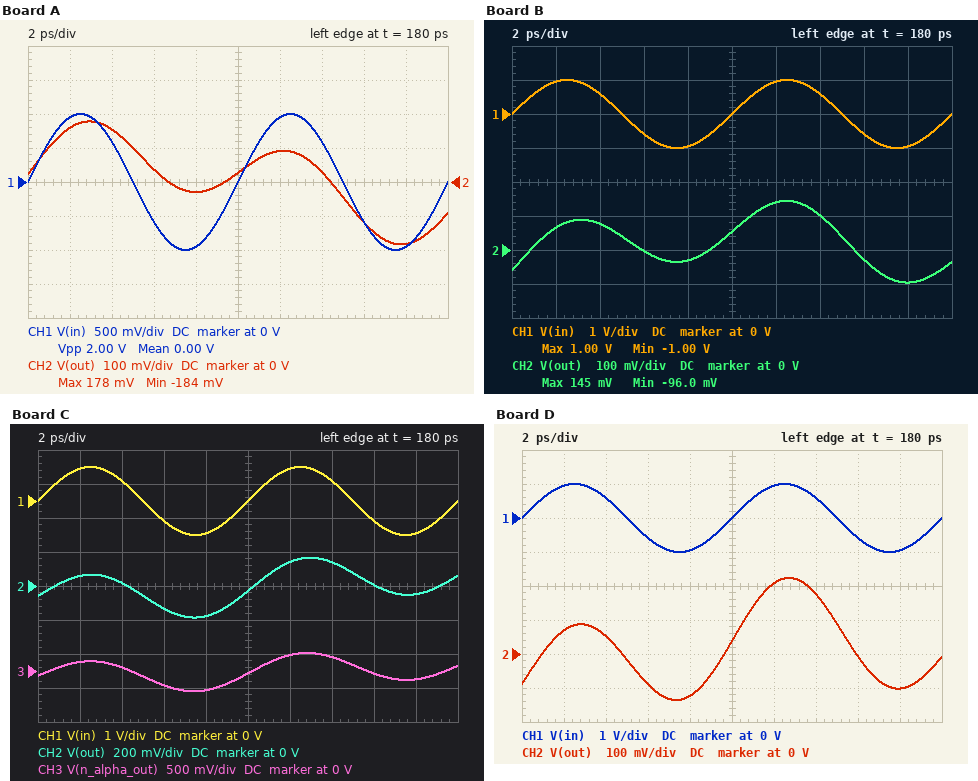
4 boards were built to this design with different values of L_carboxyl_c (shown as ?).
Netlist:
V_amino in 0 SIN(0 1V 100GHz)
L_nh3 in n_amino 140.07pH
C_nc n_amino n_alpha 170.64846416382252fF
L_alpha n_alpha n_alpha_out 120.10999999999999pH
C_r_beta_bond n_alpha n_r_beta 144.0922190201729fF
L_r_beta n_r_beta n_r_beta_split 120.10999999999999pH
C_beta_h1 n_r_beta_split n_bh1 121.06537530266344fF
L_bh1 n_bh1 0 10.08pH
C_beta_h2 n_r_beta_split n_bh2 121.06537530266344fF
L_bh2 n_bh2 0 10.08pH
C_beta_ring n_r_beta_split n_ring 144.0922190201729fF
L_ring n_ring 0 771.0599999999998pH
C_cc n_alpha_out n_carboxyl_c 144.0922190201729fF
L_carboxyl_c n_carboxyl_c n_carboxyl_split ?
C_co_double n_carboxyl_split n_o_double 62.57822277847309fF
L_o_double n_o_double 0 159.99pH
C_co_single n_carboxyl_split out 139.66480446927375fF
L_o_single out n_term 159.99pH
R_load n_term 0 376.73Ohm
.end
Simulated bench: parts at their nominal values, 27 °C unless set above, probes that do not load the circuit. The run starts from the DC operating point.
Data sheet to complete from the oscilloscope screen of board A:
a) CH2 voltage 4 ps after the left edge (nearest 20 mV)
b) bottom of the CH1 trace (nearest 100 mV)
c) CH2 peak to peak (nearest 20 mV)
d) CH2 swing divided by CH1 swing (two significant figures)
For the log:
160 mV
-1.0 V
360 mV
0.18
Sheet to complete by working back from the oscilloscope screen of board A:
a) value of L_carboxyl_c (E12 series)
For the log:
220 pH
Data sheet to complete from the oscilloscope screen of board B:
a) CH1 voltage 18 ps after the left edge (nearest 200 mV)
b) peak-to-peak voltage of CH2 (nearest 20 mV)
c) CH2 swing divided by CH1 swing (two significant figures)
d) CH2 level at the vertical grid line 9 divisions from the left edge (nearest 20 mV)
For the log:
-1.0 V
240 mV
0.12
-100 mV
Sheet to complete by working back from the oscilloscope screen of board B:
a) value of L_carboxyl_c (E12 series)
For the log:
270 pH
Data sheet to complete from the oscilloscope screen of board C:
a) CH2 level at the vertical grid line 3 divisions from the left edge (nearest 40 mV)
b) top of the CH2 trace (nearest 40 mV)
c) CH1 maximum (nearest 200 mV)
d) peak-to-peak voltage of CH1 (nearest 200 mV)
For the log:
-120 mV
160 mV
1.0 V
2.0 V
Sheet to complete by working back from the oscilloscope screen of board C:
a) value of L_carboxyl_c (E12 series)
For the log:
100 pH
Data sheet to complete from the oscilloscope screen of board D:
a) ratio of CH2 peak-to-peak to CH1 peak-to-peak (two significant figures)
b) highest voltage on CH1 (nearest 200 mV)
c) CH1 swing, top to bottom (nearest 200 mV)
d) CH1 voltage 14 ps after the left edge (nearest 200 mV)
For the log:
0.18
1.0 V
2.0 V
600 mV
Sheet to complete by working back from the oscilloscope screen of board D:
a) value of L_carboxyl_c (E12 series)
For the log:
68 pH
